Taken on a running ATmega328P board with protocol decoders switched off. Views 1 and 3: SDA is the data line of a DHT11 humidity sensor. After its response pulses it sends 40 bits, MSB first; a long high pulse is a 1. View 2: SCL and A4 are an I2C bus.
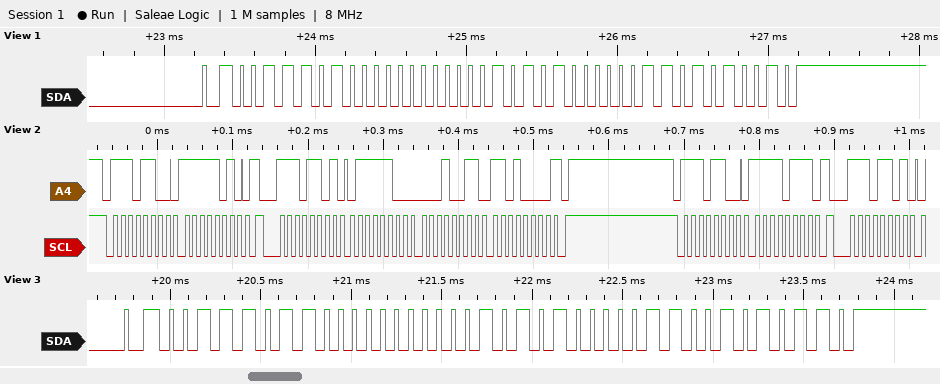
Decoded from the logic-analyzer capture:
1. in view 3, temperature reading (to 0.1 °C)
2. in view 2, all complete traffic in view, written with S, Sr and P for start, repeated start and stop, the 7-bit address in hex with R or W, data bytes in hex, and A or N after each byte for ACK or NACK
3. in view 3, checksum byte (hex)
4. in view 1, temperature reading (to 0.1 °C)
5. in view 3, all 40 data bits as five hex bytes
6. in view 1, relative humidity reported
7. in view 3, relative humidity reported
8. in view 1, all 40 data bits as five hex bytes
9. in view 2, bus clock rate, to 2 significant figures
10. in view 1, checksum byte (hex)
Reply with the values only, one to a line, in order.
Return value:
21.6 °C
S 76W A FA A Sr 76R A 7C A 13 A D0 N P S 76W A F7 A Sr 76R A
0x56
21.3 °C
3B 00 15 06 56
58 %
59 %
3A 00 15 03 52
100 kHz
0x52
